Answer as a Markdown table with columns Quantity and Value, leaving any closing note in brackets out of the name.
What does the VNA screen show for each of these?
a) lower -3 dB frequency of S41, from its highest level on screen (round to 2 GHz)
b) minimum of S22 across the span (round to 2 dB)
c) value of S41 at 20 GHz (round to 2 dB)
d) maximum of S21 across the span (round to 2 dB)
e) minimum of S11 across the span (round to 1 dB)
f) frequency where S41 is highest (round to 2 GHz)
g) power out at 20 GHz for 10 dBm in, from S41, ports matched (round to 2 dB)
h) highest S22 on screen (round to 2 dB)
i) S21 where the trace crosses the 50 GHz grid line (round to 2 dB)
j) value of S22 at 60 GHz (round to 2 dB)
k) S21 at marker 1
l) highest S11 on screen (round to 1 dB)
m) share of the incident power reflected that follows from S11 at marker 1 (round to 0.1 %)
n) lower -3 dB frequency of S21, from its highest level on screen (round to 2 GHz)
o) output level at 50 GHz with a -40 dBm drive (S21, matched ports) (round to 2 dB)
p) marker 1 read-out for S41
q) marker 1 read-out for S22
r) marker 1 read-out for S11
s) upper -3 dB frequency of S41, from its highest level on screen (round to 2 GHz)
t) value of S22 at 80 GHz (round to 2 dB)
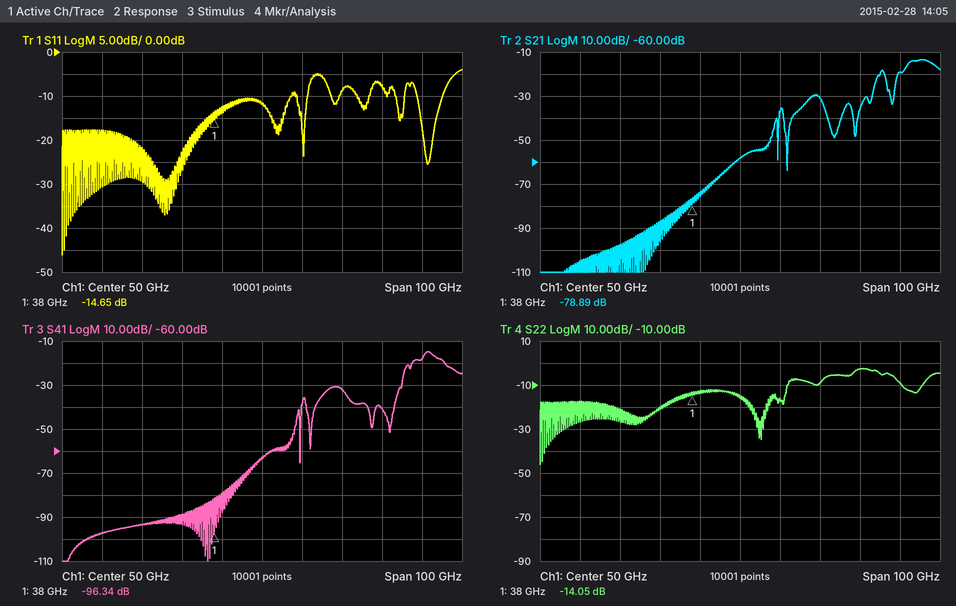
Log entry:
| Quantity | Value |
|---|---|
| lower -3 dB frequency of S41, from its highest level on screen | 90 GHz |
| minimum of S22 across the span | -46 dB |
| value of S41 at 20 GHz | -94 dB |
| maximum of S21 across the span | -14 dB |
| minimum of S11 across the span | -46 dB |
| frequency where S41 is highest | 92 GHz |
| power out at 20 GHz for 10 dBm in, from S41, ports matched | -84 dBm |
| highest S22 on screen | -2 dB |
| S21 where the trace crosses the 50 GHz grid line | -58 dB |
| value of S22 at 60 GHz | -16 dB |
| S21 at marker 1 | -78.89 dB |
| highest S11 on screen | -4 dB |
| share of the incident power reflected that follows from S11 at marker 1 | 3.4 % |
| lower -3 dB frequency of S21, from its highest level on screen | 92 GHz |
| output level at 50 GHz with a -40 dBm drive (S21, matched ports) | -98 dBm |
| marker 1 read-out for S41 | -96.34 dB |
| marker 1 read-out for S22 | -14.05 dB |
| marker 1 read-out for S11 | -14.65 dB |
| upper -3 dB frequency of S41, from its highest level on screen | 94 GHz |
| value of S22 at 80 GHz | -2 dB |
